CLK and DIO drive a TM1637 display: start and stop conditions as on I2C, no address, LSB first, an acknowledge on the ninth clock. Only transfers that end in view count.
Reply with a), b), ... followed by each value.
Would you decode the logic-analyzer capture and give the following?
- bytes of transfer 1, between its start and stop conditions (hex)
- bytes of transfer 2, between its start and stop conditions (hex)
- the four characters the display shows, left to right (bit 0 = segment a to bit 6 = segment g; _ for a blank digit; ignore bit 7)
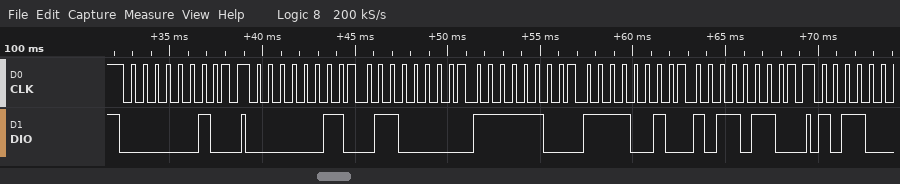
a) 40
b) C0 06 3F 4F 6D
c) 1035
